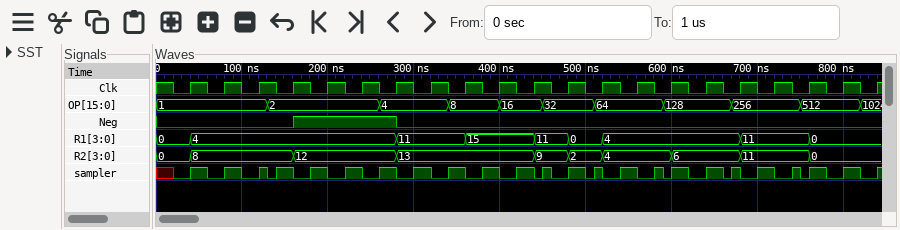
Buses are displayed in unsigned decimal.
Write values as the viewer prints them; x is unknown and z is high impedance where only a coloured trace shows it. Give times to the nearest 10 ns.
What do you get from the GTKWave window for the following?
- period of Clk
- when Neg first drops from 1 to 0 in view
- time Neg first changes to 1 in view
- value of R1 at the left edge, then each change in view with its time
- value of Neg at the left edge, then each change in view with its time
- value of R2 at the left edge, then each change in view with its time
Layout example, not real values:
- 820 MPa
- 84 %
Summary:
- 40 ns
- 280 ns
- 160 ns
- 0, 4 at 40 ns, 11 at 280 ns, 15 at 360 ns, 11 at 440 ns, 0 at 480 ns, 4 at 520 ns, 11 at 680 ns, 0 at 760 ns
- 0, 1 at 160 ns, 0 at 280 ns
- 0, 8 at 40 ns, 12 at 160 ns, 13 at 280 ns, 9 at 440 ns, 2 at 480 ns, 4 at 520 ns, 6 at 600 ns, 11 at 680 ns, 0 at 760 ns
